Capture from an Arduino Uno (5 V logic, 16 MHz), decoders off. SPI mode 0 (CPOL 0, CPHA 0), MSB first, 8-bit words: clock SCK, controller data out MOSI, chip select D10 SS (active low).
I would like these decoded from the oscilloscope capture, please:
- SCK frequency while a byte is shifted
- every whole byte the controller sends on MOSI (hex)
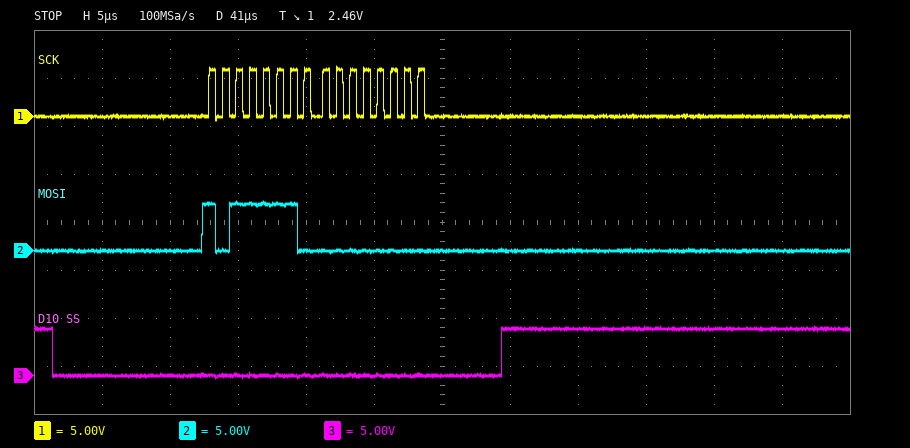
1 MHz
BE 00
